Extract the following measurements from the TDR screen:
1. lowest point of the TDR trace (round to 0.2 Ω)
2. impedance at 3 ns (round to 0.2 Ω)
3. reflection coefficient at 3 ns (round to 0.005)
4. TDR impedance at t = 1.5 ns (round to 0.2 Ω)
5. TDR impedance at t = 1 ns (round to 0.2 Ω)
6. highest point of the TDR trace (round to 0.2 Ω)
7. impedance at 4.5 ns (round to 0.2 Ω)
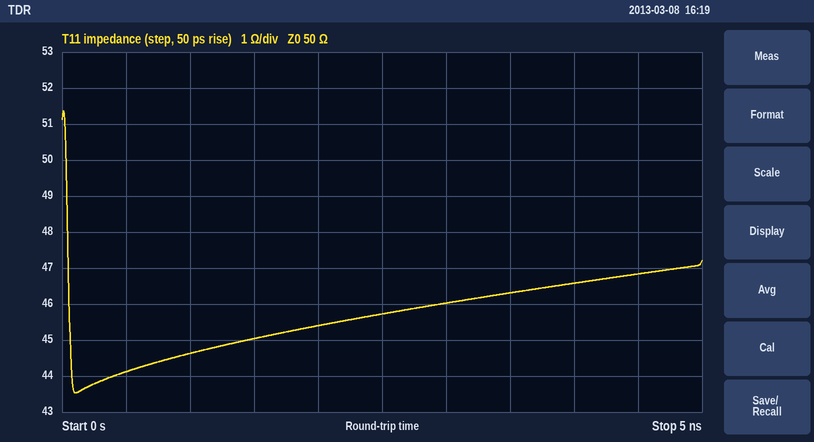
43.6 Ω
46.0 Ω
-0.040
45.0 Ω
44.6 Ω
51.4 Ω
46.8 Ω
